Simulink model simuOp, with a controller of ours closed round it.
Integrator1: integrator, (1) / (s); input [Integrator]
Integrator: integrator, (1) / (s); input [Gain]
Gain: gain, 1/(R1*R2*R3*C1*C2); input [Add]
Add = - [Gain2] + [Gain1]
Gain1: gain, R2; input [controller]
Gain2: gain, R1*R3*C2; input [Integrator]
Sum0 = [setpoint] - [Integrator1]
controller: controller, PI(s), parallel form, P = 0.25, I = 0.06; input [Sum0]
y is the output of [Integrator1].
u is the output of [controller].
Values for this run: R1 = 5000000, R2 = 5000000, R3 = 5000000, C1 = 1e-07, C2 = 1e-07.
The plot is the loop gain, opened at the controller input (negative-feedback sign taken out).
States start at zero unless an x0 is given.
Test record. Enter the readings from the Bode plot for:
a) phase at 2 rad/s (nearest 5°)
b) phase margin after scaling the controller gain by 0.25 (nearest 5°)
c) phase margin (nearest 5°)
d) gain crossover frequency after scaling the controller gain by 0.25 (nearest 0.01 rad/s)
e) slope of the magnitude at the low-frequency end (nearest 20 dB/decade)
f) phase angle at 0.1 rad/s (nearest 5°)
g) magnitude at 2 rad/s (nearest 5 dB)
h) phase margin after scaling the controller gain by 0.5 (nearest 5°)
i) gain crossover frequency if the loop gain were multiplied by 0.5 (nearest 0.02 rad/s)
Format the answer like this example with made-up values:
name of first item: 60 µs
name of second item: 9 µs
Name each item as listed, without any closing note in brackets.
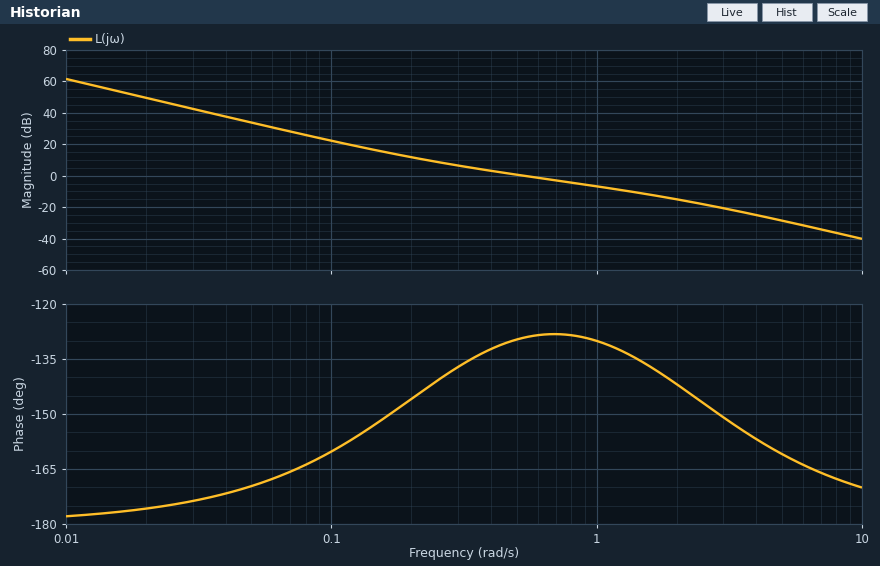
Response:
phase at 2 rad/s: -140°
phase margin after scaling the controller gain by 0.25: 35°
phase margin: 50°
gain crossover frequency after scaling the controller gain by 0.25: 0.20 rad/s
slope of the magnitude at the low-frequency end: -40 dB/decade
phase angle at 0.1 rad/s: -160°
magnitude at 2 rad/s: -15 dB
phase margin after scaling the controller gain by 0.5: 45°
gain crossover frequency if the loop gain were multiplied by 0.5: 0.32 rad/s
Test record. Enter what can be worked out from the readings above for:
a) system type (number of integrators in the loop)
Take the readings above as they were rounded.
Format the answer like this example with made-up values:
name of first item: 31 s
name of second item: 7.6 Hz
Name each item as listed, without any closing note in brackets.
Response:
system type: 2
